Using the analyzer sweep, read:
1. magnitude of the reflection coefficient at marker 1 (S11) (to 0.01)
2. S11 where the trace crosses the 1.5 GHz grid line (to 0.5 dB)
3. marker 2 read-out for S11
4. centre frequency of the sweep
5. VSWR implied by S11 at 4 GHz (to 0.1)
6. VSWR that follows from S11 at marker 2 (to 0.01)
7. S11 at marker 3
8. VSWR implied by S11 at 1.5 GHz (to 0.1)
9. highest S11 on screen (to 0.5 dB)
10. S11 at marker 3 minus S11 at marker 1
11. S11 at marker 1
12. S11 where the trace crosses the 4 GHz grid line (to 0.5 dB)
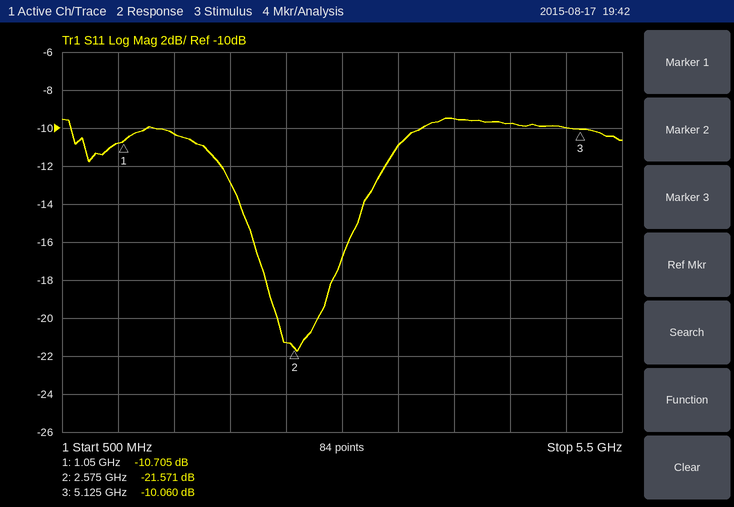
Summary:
0.29
-10.5 dB
-21.571 dB
3 GHz
2.0
1.18
-10.060 dB
1.9
-9.5 dB
0.645 dB
-10.705 dB
-9.5 dB
